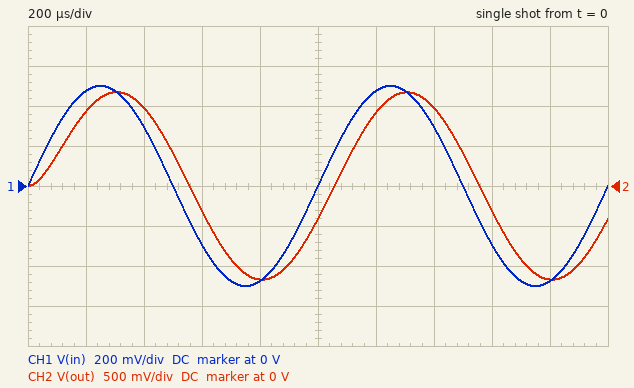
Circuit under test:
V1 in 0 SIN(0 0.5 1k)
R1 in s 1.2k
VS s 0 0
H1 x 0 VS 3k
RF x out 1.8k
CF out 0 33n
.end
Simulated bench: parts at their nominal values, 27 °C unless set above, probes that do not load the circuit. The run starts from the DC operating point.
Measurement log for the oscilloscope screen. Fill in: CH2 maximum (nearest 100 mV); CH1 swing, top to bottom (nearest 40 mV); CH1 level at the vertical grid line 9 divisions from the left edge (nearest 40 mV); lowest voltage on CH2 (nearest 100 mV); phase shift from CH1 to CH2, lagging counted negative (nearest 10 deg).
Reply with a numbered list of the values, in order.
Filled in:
1. 1.2 V
2. 1.00 V
3. -480 mV
4. -1.2 V
5. -20 deg
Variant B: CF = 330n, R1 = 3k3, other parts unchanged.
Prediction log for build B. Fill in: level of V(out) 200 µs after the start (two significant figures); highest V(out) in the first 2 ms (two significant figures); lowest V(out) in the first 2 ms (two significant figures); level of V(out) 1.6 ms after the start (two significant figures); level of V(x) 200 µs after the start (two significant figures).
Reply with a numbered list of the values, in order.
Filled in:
1. 75 mV
2. 170 mV
3. -110 mV
4. 82 mV
5. 430 mV
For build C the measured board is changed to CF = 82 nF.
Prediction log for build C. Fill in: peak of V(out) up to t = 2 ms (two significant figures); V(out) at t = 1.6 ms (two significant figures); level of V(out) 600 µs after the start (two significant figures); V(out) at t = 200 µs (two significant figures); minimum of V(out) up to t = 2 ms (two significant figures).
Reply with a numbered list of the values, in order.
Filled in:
1. 970 mV
2. 110 mV
3. 120 mV
4. 610 mV
5. -920 mV
